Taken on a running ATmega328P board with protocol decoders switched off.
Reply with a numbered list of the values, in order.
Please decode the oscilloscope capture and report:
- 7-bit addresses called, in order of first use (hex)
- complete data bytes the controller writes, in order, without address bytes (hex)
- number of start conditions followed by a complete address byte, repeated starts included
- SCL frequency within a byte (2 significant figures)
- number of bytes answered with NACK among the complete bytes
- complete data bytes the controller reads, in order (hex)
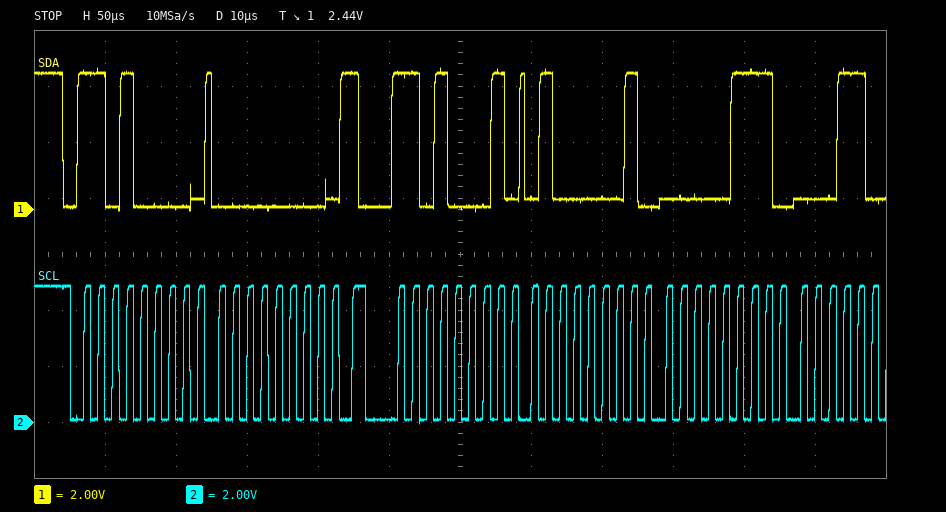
1. 0x68
2. 00
3. 2
4. 100 kHz
5. 0
6. 41 07
